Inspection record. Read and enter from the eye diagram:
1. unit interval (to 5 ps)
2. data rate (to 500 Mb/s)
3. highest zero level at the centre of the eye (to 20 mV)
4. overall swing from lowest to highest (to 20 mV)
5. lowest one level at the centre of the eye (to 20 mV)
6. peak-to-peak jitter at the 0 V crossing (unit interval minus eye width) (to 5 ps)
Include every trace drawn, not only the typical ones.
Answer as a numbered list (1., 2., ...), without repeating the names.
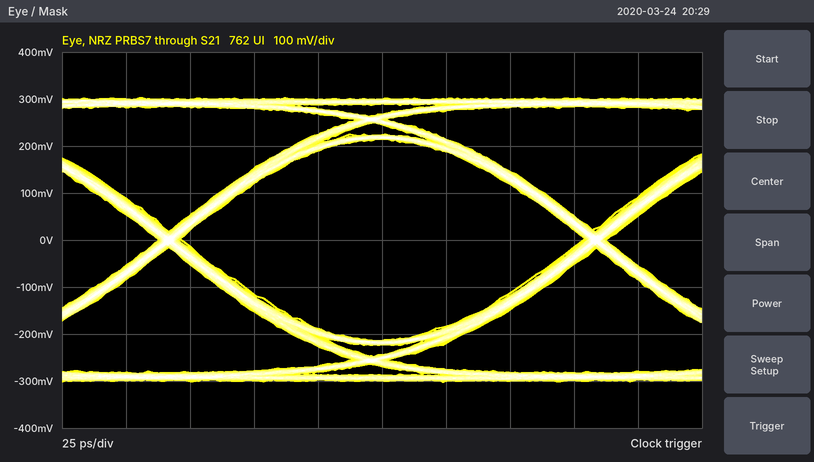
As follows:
1. 165 ps
2. 6.0 Gb/s
3. -220 mV
4. 600 mV
5. 220 mV
6. 10 ps
